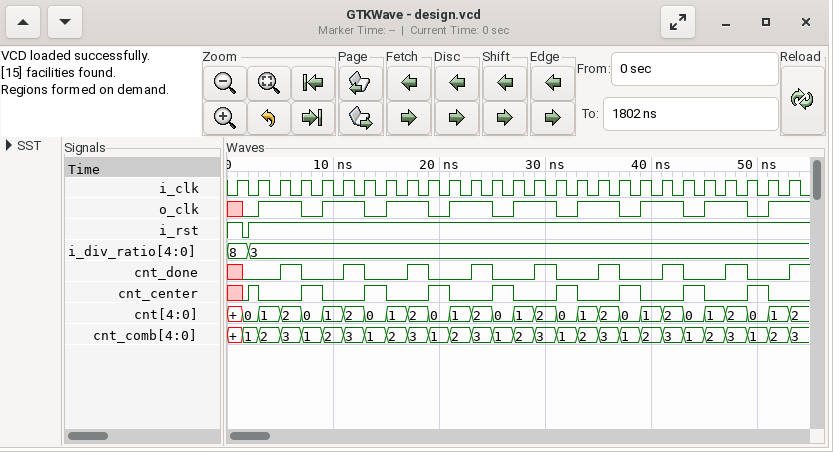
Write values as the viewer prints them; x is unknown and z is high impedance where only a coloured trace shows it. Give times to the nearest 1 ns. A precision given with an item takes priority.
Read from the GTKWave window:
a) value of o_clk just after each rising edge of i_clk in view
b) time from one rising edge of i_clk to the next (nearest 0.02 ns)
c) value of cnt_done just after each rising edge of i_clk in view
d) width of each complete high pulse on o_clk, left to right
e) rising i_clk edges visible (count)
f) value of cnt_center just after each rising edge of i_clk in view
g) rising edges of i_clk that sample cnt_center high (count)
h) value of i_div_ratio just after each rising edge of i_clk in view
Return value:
x 1 1 0 1 1 0 1 1 0 1 1 0 1 1 0 1 1 0 1 1 0 1 1 0 1 1
2 ns
x 0 1 0 0 1 0 0 1 0 0 1 0 0 1 0 0 1 0 0 1 0 0 1 0 0 1
4 ns, 4 ns, 4 ns, 4 ns, 4 ns, 4 ns, 4 ns, 4 ns
27
x 0 0 1 0 0 1 0 0 1 0 0 1 0 0 1 0 0 1 0 0 1 0 0 1 0 0
9
8, 3, 3, 3, 3, 3, 3, 3, 3, 3, 3, 3, 3, 3, 3, 3, 3, 3, 3, 3, 3, 3, 3, 3, 3, 3, 3
